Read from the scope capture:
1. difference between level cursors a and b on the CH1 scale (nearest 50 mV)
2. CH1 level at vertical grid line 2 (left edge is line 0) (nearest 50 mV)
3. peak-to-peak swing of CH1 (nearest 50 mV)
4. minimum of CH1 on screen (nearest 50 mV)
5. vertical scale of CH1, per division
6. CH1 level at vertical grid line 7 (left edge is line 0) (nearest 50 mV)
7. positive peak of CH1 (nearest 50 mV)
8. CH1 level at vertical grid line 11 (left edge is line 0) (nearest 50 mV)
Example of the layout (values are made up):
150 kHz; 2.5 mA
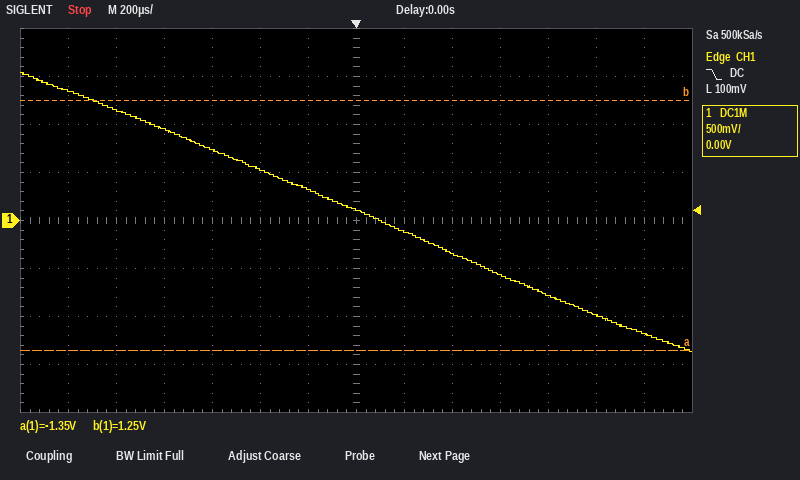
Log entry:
2.60 V; 1.15 V; 2.90 V; -1.35 V; 500 mV; 100 mV; 1.55 V; -800 mV
